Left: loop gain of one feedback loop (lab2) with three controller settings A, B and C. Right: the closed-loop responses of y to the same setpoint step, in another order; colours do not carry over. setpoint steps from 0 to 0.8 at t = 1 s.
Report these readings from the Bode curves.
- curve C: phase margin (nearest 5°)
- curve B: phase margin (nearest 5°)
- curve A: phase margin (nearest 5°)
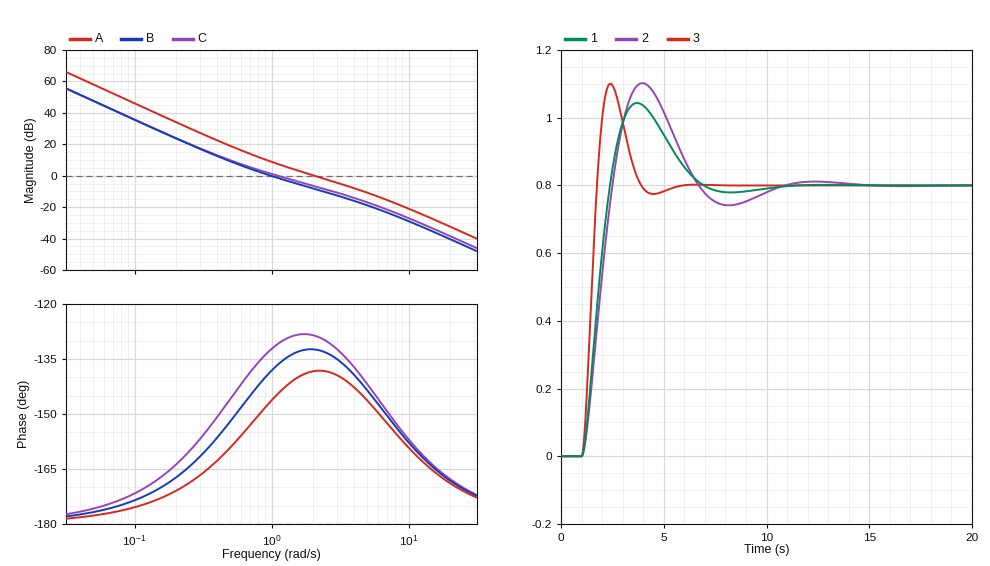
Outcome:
50°
40°
40°
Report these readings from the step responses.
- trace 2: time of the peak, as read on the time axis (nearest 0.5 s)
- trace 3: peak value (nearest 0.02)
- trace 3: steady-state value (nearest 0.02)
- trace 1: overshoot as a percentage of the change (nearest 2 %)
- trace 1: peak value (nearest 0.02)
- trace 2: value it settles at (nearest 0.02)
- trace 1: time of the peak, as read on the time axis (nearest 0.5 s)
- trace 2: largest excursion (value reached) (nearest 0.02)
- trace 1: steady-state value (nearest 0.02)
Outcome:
4.0 s
1.10
0.80
30 %
1.04
0.80
3.5 s
1.10
0.80
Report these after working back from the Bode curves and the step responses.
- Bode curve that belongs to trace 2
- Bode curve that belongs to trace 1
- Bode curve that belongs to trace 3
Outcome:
B
C
A
